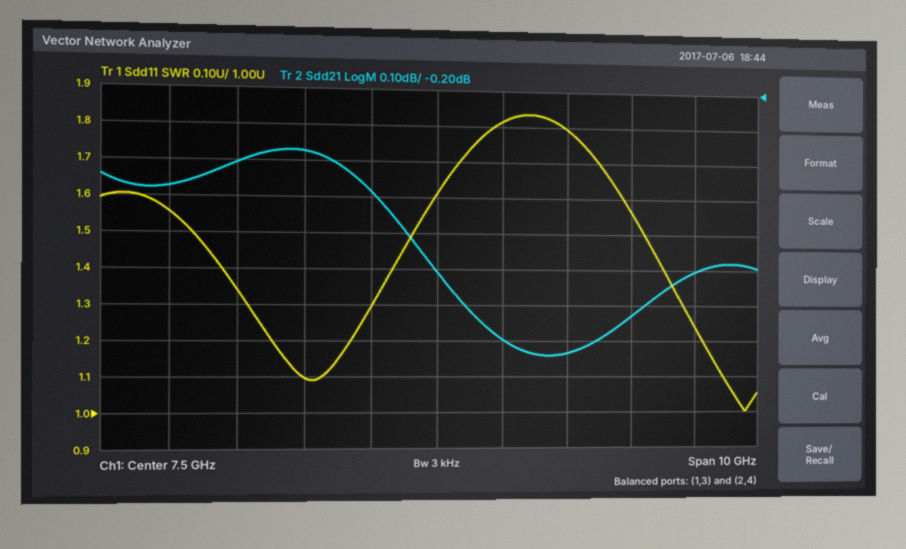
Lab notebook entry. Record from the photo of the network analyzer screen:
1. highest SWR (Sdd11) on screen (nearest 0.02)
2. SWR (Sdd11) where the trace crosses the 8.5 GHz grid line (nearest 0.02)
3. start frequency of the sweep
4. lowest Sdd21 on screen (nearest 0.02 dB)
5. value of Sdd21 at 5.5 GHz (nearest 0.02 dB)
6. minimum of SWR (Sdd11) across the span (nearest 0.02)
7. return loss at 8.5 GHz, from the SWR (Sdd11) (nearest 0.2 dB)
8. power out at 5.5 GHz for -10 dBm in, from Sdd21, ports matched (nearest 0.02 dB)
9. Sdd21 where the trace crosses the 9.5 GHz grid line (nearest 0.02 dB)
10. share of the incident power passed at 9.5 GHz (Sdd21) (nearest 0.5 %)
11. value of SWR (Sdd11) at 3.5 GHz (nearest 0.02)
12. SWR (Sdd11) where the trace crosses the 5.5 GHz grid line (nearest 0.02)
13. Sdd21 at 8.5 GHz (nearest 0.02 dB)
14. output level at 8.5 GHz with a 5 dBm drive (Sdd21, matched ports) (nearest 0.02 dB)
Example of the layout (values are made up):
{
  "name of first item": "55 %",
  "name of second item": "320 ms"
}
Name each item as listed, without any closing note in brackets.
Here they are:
{
  "highest SWR (Sdd11) on screen": "1.84",
  "SWR (Sdd11) where the trace crosses the 8.5 GHz grid line": "1.82",
  "start frequency of the sweep": "2.5 GHz",
  "lowest Sdd21 on screen": "-0.94 dB",
  "value of Sdd21 at 5.5 GHz": "-0.38 dB",
  "minimum of SWR (Sdd11) across the span": "1.00",
  "return loss at 8.5 GHz, from the SWR (Sdd11)": "10.8 dB",
  "power out at 5.5 GHz for -10 dBm in, from Sdd21, ports matched": "-10.38 dBm",
  "Sdd21 where the trace crosses the 9.5 GHz grid line": "-0.94 dB",
  "share of the incident power passed at 9.5 GHz (Sdd21)": "80.5 %",
  "value of SWR (Sdd11) at 3.5 GHz": "1.56",
  "SWR (Sdd11) where the trace crosses the 5.5 GHz grid line": "1.10",
  "Sdd21 at 8.5 GHz": "-0.90 dB",
  "output level at 8.5 GHz with a 5 dBm drive (Sdd21, matched ports)": "4.10 dBm"
}
